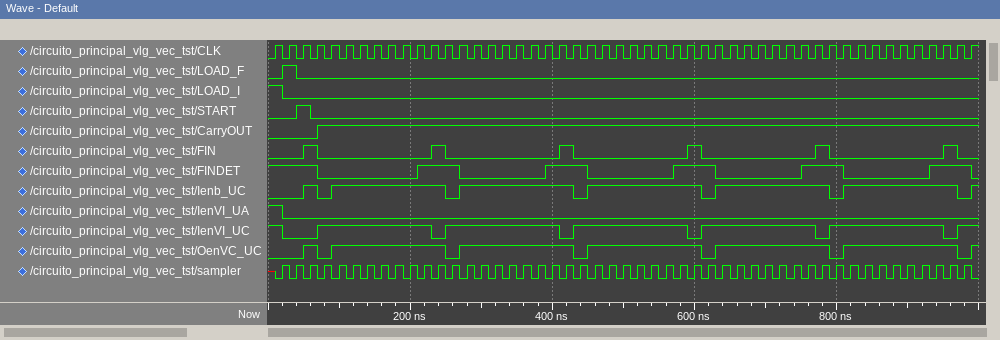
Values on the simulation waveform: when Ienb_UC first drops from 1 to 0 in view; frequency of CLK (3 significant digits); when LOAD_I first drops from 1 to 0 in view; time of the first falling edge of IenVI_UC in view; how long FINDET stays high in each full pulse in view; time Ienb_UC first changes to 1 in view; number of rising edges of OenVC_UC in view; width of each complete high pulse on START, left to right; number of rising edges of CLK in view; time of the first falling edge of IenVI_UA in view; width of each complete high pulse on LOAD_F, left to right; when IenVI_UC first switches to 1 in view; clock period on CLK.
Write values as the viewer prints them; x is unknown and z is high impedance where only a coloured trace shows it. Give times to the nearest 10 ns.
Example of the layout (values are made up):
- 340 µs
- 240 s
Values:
- 70 ns
- 50.0 MHz
- 20 ns
- 20 ns
- 60 ns, 60 ns, 60 ns, 60 ns, 60 ns
- 50 ns
- 7
- 20 ns
- 50
- 20 ns
- 20 ns
- 70 ns
- 20 ns
